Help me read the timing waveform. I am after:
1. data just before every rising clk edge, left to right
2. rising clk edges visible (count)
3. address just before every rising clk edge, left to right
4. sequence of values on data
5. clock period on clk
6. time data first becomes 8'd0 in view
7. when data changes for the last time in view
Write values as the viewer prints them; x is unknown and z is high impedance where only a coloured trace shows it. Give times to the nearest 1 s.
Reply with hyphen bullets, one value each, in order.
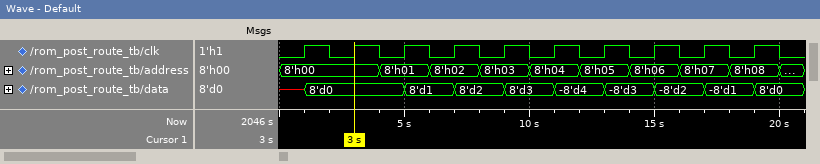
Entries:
- x, 8'd0, 8'd0, 8'd1, 8'd2, 8'd3, -8'd4, -8'd3, -8'd2, -8'd1
- 10
- 8'h00, 8'h00, 8'h01, 8'h02, 8'h03, 8'h04, 8'h05, 8'h06, 8'h07, 8'h08
- x, 8'd0, 8'd1, 8'd2, 8'd3, -8'd4, -8'd3, -8'd2, -8'd1, 8'd0
- 2 s
- 1 s
- 19 s
